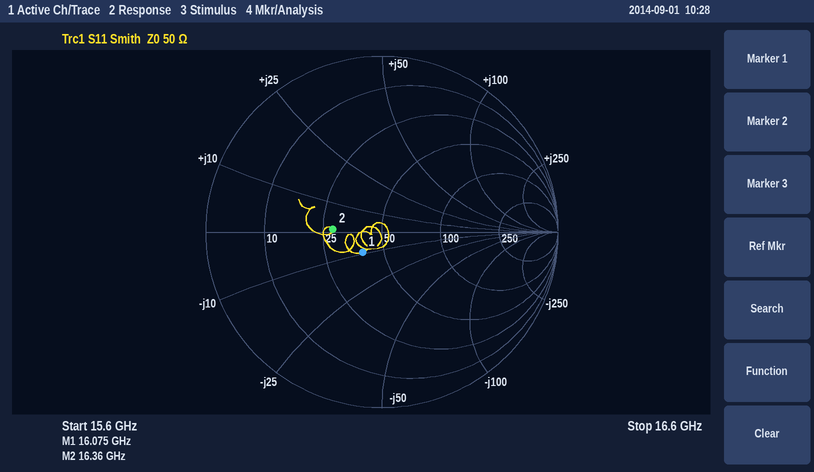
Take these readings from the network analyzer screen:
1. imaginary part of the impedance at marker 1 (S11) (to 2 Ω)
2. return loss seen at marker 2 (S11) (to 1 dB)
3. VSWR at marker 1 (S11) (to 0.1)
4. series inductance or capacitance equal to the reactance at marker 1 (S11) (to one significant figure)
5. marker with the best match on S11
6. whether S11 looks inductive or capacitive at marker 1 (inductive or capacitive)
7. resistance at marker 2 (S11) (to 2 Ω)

-10 Ω
11 dB
1.4
1 pF
marker 1
capacitive
28 Ω
